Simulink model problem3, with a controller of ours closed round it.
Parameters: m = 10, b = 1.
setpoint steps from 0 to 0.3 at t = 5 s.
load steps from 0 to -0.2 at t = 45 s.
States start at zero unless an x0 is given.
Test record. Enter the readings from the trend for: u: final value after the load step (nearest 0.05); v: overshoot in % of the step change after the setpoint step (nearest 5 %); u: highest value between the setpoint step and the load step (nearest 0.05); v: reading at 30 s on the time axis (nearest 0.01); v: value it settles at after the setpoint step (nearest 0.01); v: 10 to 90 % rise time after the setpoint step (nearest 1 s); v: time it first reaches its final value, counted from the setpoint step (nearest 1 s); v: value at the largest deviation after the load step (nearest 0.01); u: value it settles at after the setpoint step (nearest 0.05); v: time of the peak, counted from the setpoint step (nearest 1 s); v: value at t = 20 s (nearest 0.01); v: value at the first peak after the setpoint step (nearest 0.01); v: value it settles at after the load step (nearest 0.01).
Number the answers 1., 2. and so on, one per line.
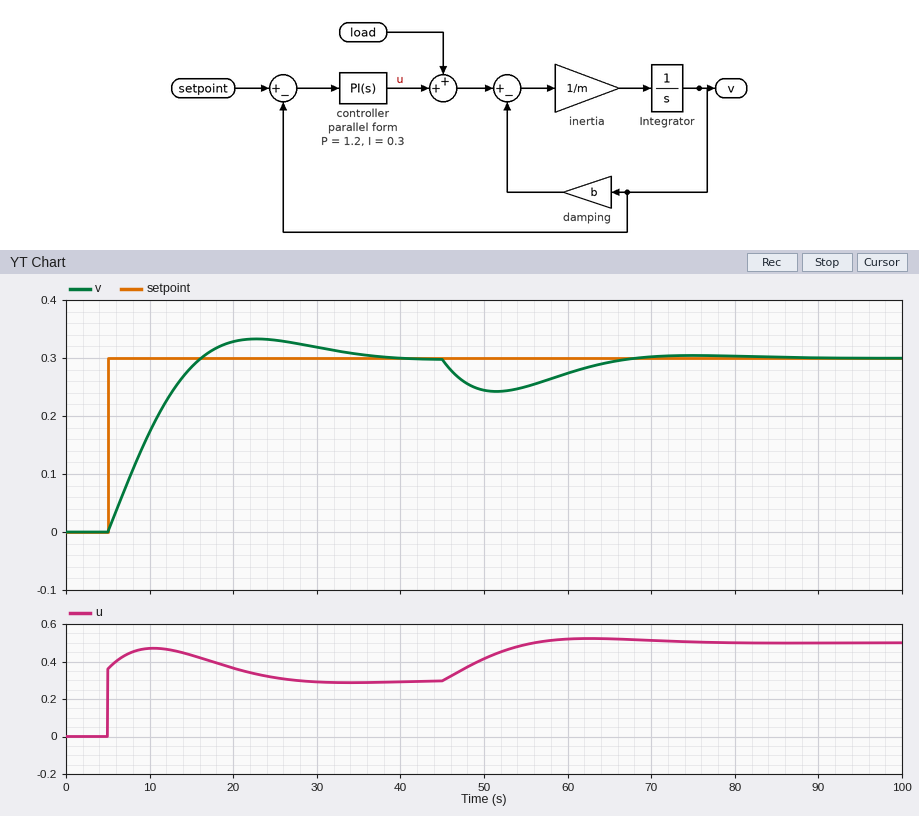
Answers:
1. 0.50
2. 10 %
3. 0.45
4. 0.32
5. 0.30
6. 8 s
7. 11 s
8. 0.24
9. 0.30
10. 18 s
11. 0.33
12. 0.33
13. 0.30
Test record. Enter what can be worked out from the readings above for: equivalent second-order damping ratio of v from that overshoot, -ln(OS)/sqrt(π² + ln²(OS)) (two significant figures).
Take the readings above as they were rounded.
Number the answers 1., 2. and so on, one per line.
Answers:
1. 0.59
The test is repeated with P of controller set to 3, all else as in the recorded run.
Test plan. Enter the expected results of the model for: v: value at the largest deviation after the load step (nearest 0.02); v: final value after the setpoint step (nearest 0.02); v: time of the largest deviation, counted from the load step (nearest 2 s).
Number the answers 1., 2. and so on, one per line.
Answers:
1. 0.26
2. 0.30
3. 6 s
